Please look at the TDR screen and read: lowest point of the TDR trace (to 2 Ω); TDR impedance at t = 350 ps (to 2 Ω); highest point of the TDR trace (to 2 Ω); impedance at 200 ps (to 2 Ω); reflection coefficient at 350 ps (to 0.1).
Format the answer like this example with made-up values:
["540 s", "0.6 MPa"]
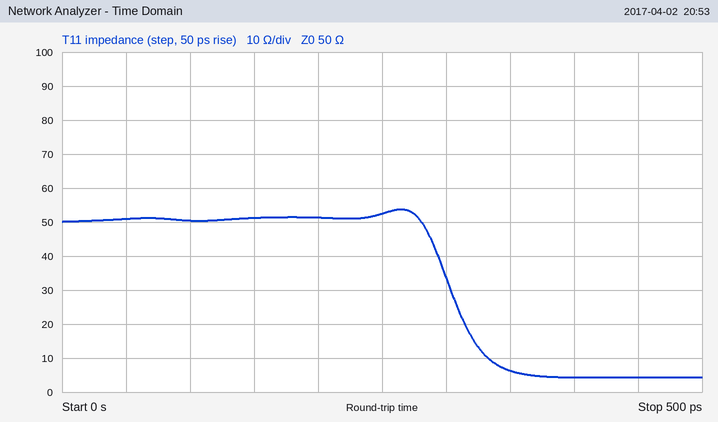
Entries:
["4 Ω", "6 Ω", "54 Ω", "52 Ω", "-0.8"]
